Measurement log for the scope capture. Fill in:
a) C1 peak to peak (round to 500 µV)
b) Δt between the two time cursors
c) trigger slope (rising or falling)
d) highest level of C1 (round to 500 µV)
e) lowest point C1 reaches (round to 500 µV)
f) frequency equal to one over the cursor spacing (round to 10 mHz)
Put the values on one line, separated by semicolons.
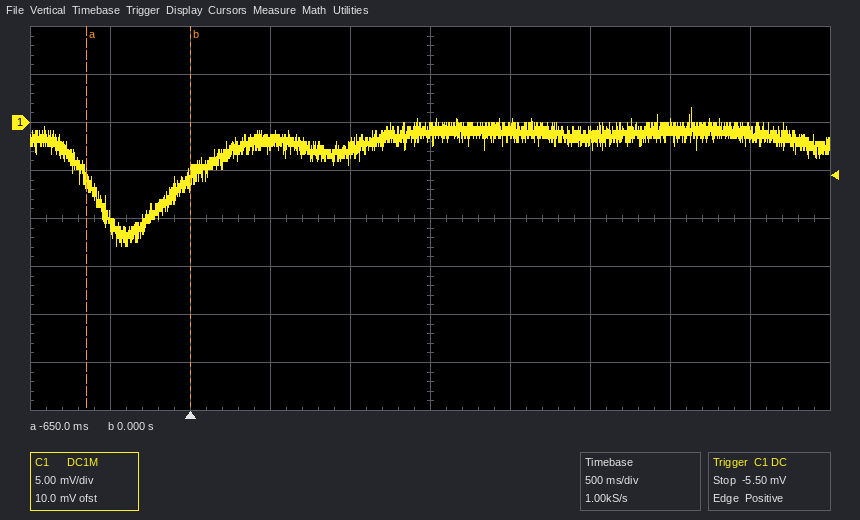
14.5 mV; 650 ms; rising; 1.5 mV; -13.0 mV; 1.54 Hz
